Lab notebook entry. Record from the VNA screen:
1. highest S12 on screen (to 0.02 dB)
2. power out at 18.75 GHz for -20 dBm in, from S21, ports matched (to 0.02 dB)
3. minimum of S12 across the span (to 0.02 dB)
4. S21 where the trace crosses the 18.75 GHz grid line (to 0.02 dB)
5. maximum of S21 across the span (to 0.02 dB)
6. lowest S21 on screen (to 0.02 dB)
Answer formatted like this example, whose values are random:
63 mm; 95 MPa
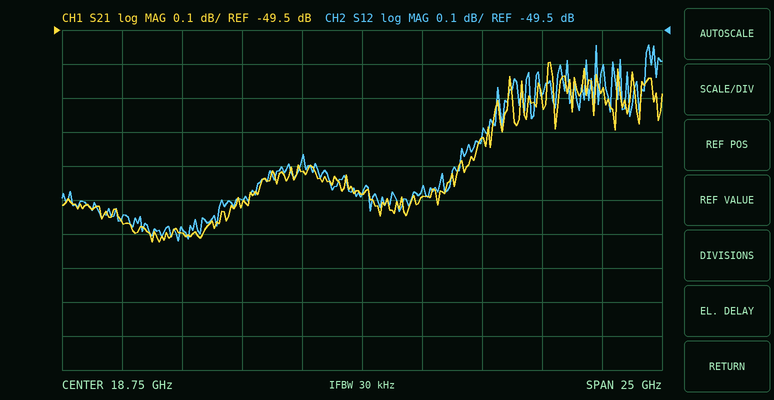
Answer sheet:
-49.54 dB; -69.98 dBm; -50.12 dB; -49.98 dB; -49.60 dB; -50.12 dB
